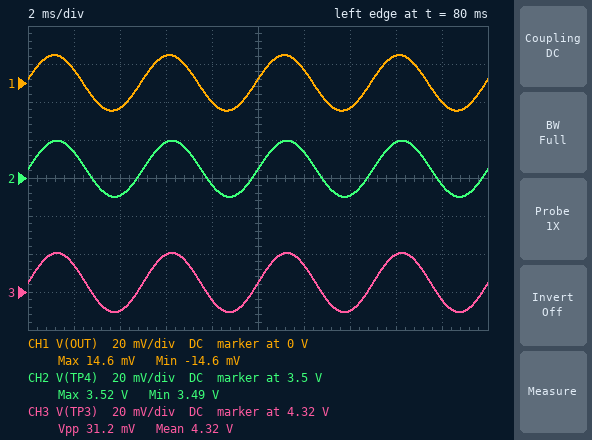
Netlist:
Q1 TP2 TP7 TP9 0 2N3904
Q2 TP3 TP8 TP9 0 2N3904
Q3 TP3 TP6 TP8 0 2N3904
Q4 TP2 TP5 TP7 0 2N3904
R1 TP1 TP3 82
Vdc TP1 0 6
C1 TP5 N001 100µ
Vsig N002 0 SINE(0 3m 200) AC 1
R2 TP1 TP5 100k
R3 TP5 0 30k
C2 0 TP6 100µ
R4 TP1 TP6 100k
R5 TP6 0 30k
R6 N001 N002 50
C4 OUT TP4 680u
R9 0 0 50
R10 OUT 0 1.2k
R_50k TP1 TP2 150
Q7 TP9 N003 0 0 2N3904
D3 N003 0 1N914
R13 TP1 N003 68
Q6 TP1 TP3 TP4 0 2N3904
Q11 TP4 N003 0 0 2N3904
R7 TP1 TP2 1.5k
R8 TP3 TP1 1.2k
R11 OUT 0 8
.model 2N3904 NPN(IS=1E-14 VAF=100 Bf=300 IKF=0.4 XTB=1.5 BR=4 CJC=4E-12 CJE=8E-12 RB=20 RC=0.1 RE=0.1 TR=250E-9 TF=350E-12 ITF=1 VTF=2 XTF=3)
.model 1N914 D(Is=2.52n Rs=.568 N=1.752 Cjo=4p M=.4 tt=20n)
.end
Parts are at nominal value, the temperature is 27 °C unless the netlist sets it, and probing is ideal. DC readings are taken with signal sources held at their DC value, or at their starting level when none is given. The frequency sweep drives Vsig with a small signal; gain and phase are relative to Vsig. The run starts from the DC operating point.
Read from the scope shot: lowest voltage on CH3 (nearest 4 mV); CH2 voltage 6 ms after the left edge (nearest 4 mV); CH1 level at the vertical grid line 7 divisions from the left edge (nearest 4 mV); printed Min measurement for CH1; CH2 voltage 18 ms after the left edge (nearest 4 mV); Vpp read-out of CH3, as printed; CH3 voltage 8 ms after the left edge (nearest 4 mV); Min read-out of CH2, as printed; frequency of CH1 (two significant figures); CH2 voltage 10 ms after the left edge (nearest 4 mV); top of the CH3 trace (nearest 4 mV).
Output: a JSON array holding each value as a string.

["4.308 V", "3.520 V", "-12 mV", "-14.6 mV", "3.496 V", "31.2 mV", "4.316 V", "3.49 V", "200 Hz", "3.504 V", "4.340 V"]
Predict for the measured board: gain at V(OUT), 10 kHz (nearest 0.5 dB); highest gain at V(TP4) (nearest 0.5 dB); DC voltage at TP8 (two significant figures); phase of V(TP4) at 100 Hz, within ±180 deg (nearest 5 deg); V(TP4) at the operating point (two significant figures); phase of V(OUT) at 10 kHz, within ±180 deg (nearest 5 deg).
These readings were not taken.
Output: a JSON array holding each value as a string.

["14.0 dB", "14.5 dB", "790 mV", "0 deg", "3.5 V", "0 deg"]
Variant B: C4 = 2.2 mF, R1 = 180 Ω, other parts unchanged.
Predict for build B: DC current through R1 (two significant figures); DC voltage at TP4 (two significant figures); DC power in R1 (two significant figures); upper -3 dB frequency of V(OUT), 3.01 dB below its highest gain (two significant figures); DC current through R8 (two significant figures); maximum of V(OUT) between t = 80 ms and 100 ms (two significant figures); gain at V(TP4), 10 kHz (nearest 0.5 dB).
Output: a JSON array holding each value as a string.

["19 mA", "1.8 V", "62 mW", "770 kHz", "2.8 mA", "28 mV", "19.5 dB"]
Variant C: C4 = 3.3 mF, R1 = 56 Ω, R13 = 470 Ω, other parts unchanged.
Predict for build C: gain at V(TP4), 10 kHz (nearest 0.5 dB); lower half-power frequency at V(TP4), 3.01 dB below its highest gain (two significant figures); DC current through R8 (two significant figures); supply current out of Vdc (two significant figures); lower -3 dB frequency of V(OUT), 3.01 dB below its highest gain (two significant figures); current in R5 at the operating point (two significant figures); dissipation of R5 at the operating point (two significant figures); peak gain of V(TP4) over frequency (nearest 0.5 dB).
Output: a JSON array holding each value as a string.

["-1.5 dB", "68 mHz", "120 µA", "22 mA", "3.7 Hz", "46 µA", "64 µW", "2.5 dB"]
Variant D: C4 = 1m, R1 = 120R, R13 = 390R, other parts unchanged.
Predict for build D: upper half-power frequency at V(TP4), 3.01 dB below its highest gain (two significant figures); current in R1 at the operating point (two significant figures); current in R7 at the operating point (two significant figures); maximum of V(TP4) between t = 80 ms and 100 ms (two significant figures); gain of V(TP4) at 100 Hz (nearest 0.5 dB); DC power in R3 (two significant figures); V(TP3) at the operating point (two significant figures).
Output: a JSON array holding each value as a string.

["48 Hz", "3.5 mA", "350 µA", "4.9 V", "8.5 dB", "64 µW", "5.6 V"]
